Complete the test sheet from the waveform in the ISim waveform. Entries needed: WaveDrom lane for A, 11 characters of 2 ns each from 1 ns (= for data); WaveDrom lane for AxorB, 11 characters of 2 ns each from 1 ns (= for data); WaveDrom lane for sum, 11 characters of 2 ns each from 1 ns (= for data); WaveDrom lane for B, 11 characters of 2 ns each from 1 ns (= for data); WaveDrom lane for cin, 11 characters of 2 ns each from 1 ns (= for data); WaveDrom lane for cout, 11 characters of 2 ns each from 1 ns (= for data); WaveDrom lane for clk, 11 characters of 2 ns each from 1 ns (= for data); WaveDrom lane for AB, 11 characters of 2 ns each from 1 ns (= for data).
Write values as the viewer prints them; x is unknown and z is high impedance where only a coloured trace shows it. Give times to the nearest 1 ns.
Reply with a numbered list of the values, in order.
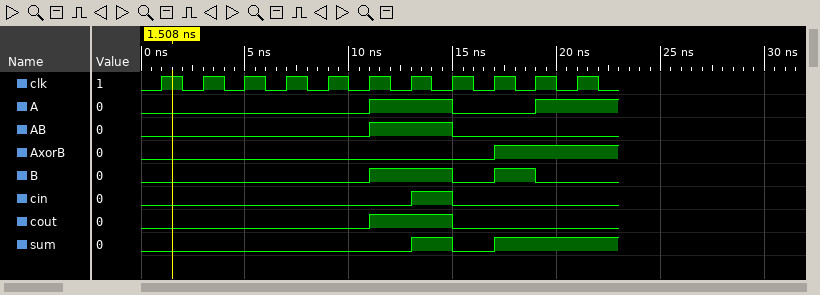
1. {name: 'A', wave: '0....1.0.1.'}
2. {name: 'AxorB', wave: '0.......1..'}
3. {name: 'sum', wave: '0.....101..'}
4. {name: 'B', wave: '0....1.010.'}
5. {name: 'cin', wave: '0.....10...'}
6. {name: 'cout', wave: '0....1.0...'}
7. {name: 'clk', wave: 'p..........'}
8. {name: 'AB', wave: '0....1.0...'}
